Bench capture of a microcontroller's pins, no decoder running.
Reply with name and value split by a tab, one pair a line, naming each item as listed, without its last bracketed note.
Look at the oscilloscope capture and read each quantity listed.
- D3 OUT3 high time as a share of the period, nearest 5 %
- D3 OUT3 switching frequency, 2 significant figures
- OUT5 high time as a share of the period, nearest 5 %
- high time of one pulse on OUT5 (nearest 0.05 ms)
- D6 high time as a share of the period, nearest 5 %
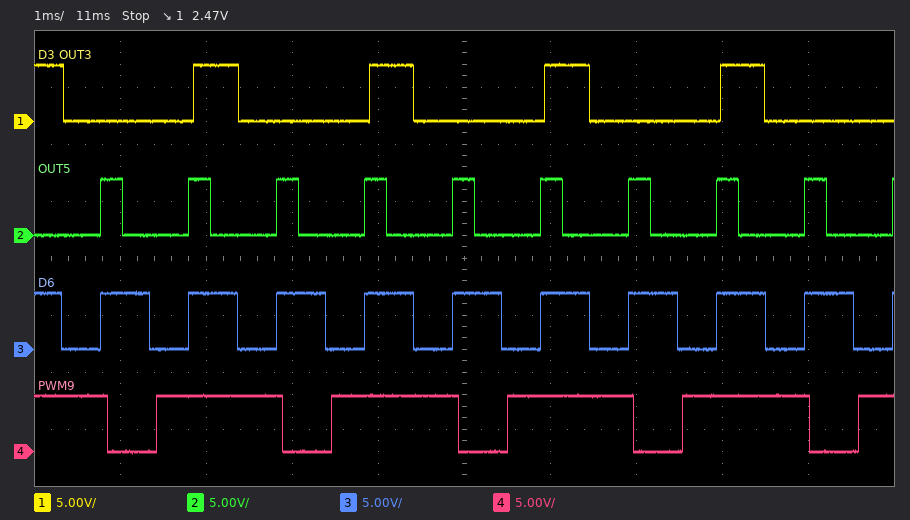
D3 OUT3 high time as a share of the period, nearest 5 %	25 %
D3 OUT3 switching frequency, 2 significant figures	490 Hz
OUT5 high time as a share of the period, nearest 5 %	25 %
high time of one pulse on OUT5	0.25 ms
D6 high time as a share of the period, nearest 5 %	55 %
